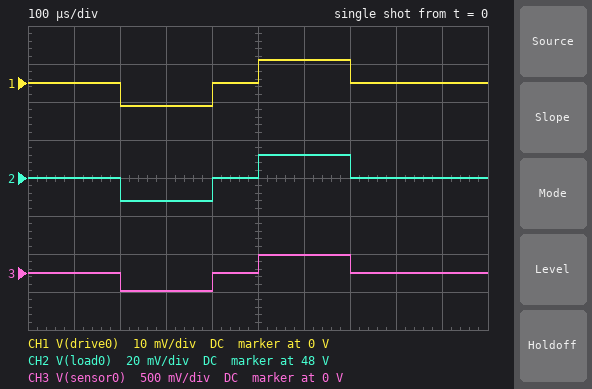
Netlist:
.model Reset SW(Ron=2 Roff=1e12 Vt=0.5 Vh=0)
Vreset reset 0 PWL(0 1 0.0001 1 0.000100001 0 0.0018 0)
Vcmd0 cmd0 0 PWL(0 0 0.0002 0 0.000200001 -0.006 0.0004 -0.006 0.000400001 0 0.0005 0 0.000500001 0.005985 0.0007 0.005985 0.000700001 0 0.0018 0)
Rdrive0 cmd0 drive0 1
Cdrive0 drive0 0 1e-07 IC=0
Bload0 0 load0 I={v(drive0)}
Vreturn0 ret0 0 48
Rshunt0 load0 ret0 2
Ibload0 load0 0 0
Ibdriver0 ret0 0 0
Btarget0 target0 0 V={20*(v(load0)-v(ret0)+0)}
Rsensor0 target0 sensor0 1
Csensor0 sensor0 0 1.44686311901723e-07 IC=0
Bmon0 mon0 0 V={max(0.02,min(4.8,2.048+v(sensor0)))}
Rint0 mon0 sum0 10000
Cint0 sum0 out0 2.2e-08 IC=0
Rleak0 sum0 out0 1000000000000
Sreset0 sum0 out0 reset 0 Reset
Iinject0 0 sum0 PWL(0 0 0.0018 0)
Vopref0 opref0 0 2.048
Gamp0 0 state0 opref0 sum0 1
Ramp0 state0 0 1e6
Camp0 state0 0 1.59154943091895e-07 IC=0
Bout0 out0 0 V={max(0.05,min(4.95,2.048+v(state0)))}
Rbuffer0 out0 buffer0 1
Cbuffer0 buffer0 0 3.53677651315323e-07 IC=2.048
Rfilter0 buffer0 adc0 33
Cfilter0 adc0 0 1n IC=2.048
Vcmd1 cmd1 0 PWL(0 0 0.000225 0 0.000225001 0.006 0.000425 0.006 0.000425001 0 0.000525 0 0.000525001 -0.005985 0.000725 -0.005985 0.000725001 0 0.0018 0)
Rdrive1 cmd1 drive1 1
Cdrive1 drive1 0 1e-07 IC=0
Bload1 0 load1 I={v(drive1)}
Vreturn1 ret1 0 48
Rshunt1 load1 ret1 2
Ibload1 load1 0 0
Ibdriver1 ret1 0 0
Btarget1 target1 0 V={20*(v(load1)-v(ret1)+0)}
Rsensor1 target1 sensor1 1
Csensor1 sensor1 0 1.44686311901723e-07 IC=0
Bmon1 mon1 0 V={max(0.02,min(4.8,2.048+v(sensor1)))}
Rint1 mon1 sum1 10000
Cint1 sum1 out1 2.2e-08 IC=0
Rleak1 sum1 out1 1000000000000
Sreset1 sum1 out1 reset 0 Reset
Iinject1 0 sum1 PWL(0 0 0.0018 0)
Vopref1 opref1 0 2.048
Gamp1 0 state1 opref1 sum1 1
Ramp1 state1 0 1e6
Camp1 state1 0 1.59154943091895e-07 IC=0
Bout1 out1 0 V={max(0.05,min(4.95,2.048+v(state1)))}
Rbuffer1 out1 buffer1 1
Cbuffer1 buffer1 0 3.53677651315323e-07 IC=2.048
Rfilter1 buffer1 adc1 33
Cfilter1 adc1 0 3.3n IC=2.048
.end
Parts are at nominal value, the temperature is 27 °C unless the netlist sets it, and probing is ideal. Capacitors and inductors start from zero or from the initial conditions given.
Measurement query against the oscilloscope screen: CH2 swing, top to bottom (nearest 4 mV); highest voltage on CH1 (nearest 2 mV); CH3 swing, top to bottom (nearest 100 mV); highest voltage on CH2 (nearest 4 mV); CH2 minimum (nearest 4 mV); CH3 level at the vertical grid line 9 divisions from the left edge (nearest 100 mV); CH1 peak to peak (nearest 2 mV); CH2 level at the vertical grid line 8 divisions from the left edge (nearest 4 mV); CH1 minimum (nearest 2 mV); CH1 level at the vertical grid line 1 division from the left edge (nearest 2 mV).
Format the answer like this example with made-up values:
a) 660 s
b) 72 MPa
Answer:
a) 24 mV
b) 6 mV
c) 500 mV
d) 48.012 V
e) 47.988 V
f) 0 V
g) 12 mV
h) 48.000 V
i) -6 mV
j) 0 V
